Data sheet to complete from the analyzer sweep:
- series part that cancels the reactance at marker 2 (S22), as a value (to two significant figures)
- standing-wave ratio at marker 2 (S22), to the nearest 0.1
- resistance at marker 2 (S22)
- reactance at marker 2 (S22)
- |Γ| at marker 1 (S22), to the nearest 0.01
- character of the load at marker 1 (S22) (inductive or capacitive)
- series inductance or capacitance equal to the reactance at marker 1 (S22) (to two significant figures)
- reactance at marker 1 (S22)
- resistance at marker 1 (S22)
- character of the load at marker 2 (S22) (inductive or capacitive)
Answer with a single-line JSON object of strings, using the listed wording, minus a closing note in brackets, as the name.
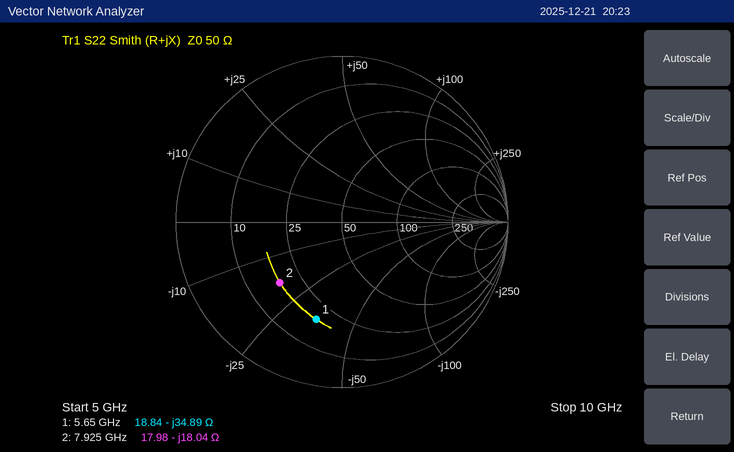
{"series part that cancels the reactance at marker 2 (S22), as a value": "360 pH", "standing-wave ratio at marker 2 (S22), to the nearest 0.1": "3.2", "resistance at marker 2": "17.98 Ω", "reactance at marker 2": "-18.04 Ω", "|Γ| at marker 1 (S22), to the nearest 0.01": "0.61", "character of the load at marker 1 (S22)": "capacitive", "series inductance or capacitance equal to the reactance at marker 1 (S22)": "810 fF", "reactance at marker 1": "-34.89 Ω", "resistance at marker 1": "18.84 Ω", "character of the load at marker 2 (S22)": "capacitive"}
